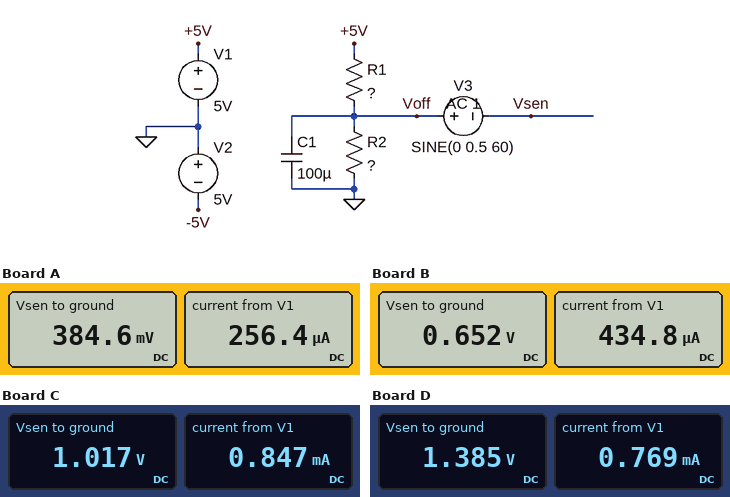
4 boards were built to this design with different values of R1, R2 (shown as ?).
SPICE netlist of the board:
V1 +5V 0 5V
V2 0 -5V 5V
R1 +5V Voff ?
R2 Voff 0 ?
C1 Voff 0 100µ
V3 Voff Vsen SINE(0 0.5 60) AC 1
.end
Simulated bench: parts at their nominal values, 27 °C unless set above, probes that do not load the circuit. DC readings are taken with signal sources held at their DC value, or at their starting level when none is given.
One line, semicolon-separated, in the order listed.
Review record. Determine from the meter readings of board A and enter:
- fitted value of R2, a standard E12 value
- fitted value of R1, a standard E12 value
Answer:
1.5 kΩ; 18 kΩ
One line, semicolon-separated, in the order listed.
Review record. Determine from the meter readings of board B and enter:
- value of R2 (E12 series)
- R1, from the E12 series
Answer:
1.5 kΩ; 10 kΩ
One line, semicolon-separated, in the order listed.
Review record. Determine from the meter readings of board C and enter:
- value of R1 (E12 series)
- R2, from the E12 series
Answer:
4.7 kΩ; 1.2 kΩ
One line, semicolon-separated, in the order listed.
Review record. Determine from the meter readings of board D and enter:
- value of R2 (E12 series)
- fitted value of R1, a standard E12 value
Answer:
1.8 kΩ; 4.7 kΩ
